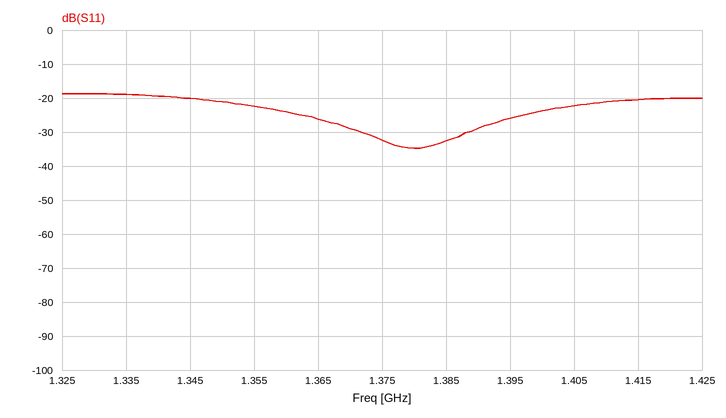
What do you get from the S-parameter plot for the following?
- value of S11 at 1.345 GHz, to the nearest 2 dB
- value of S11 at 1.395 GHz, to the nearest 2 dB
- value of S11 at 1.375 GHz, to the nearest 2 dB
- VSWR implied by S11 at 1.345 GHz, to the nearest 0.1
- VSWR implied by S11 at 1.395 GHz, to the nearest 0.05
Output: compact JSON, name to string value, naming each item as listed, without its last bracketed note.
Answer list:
{"value of S11 at 1.345 GHz, to the nearest 2 dB": "-20 dB", "value of S11 at 1.395 GHz, to the nearest 2 dB": "-26 dB", "value of S11 at 1.375 GHz, to the nearest 2 dB": "-32 dB", "VSWR implied by S11 at 1.345 GHz, to the nearest 0.1": "1.2", "VSWR implied by S11 at 1.395 GHz, to the nearest 0.05": "1.10"}
